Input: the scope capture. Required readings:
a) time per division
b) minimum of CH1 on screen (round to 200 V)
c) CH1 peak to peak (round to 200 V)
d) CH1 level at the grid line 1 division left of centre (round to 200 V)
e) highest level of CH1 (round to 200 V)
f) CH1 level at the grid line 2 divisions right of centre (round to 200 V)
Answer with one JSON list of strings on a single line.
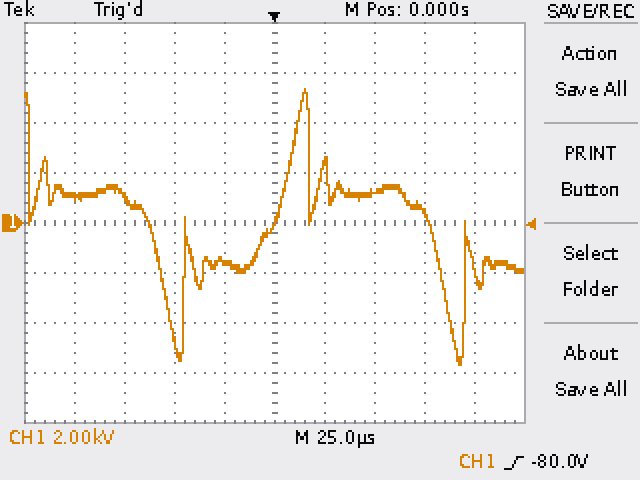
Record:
["25 µs", "-5.6 kV", "11.0 kV", "-1.6 kV", "5.4 kV", "1.2 kV"]
